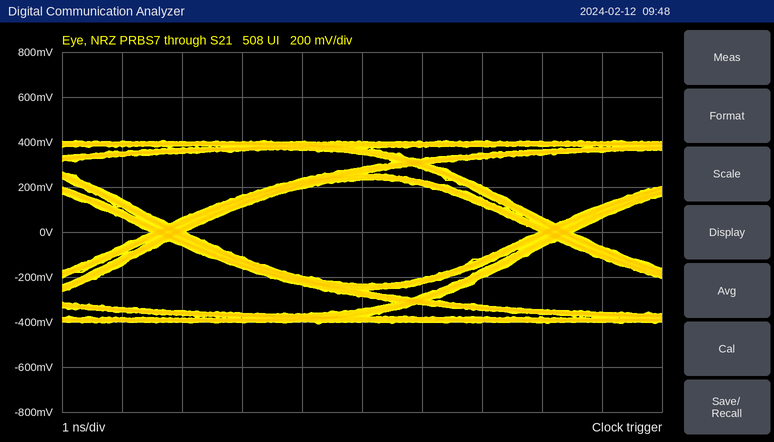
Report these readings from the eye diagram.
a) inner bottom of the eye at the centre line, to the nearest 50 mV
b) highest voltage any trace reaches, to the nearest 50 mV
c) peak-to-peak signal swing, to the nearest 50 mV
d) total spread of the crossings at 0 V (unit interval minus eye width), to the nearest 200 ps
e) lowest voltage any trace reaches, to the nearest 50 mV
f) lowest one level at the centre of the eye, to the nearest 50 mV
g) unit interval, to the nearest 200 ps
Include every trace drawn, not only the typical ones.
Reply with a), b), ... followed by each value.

a) -250 mV
b) 400 mV
c) 800 mV
d) 600 ps
e) -400 mV
f) 250 mV
g) 6.4 ns
